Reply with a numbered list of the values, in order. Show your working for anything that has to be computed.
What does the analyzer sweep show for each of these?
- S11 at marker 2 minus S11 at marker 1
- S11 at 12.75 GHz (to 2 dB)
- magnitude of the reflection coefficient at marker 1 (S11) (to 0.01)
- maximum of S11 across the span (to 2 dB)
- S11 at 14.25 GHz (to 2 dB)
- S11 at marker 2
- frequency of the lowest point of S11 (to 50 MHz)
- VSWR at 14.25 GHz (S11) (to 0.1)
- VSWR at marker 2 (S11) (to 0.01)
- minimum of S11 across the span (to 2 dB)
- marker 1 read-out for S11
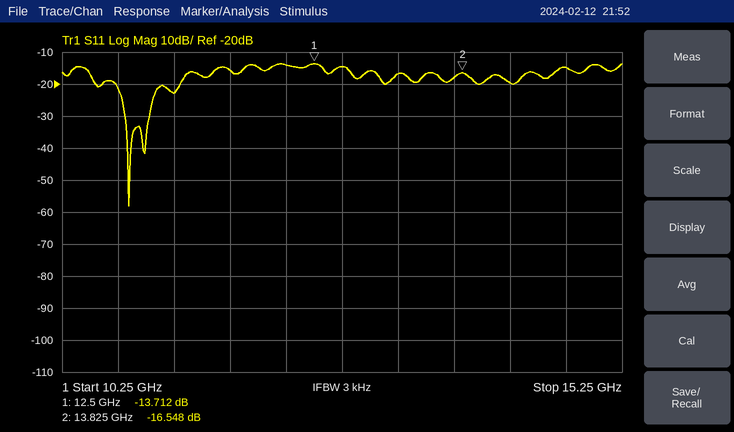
1. -16.548 − (-13.712) = -2.836 dB
2. -14 dB
3. 10^(-13.712/20) ≈ 0.21
4. -14 dB
5. -20 dB
6. -16.548 dB
7. 10.85 GHz
8. |Γ| = 10^(-20/20) = 0.1000; VSWR = (1 + 0.1000)/(1 − 0.1000) ≈ 1.2
9. (1 + 0.1488)/(1 − 0.1488) ≈ 1.35
10. -58 dB
11. -13.712 dB
